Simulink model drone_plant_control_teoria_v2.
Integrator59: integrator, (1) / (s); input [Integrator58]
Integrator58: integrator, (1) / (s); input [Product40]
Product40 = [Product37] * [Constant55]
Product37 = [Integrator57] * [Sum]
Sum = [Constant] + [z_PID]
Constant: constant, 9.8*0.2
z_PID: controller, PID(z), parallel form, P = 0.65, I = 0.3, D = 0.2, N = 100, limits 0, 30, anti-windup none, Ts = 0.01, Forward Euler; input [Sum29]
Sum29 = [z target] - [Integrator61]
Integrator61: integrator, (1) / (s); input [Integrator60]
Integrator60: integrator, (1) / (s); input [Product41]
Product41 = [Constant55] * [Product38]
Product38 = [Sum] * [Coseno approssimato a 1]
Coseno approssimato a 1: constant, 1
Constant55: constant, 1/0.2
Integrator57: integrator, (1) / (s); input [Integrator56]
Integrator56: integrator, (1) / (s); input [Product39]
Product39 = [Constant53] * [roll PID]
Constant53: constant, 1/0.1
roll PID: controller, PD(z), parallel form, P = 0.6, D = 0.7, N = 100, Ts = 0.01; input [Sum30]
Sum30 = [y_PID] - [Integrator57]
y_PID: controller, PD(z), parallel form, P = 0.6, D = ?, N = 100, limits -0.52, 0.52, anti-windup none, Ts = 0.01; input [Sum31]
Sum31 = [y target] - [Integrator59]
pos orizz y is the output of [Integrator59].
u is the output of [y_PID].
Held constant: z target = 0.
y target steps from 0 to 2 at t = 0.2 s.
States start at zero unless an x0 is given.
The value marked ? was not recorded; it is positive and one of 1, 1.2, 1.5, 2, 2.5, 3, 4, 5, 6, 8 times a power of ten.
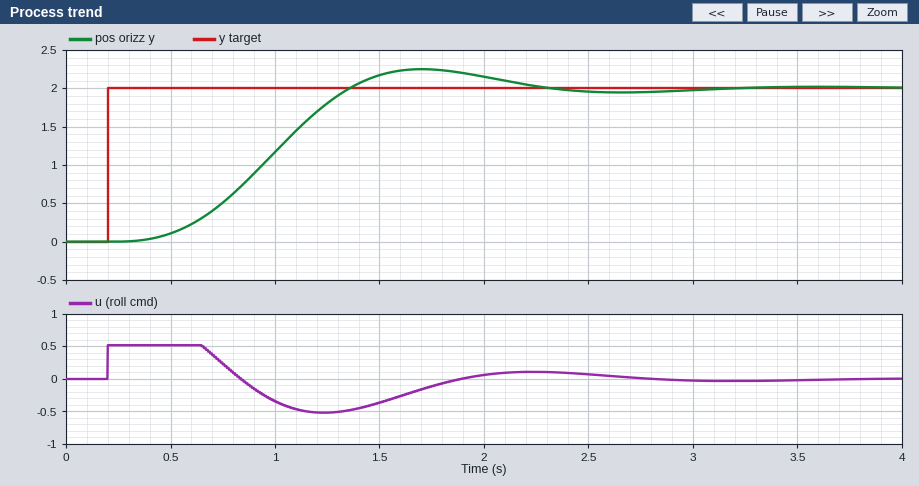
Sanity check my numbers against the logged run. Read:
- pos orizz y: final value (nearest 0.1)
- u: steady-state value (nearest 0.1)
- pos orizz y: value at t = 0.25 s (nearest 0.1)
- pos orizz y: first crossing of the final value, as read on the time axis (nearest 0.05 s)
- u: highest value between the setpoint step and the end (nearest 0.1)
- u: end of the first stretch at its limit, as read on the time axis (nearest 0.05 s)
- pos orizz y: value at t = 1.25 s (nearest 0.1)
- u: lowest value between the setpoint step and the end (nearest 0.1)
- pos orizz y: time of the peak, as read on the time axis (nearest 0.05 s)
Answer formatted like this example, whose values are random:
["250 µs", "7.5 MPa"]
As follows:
["2.0", "0.0", "0.0", "1.35 s", "0.5", "0.65 s", "1.8", "-0.5", "1.70 s"]
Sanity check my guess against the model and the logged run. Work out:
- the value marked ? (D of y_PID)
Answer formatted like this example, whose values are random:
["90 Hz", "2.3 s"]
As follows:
["0.3"]
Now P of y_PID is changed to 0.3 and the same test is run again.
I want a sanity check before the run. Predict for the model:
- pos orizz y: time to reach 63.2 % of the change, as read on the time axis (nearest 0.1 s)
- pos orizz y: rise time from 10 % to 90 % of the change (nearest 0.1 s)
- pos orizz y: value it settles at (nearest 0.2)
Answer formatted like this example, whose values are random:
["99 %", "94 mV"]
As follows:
["1.3 s", "1.4 s", "2.0"]
